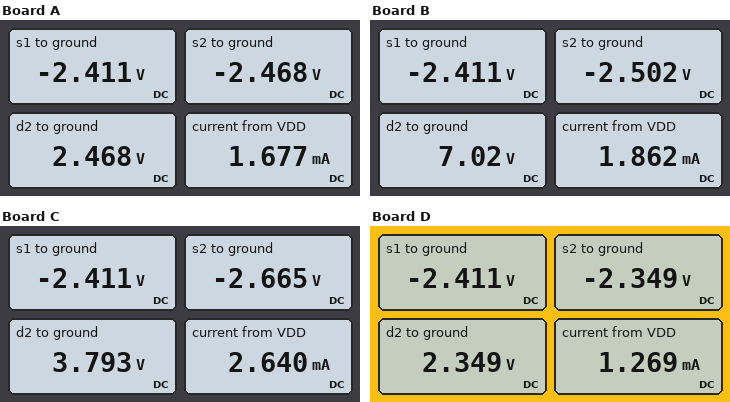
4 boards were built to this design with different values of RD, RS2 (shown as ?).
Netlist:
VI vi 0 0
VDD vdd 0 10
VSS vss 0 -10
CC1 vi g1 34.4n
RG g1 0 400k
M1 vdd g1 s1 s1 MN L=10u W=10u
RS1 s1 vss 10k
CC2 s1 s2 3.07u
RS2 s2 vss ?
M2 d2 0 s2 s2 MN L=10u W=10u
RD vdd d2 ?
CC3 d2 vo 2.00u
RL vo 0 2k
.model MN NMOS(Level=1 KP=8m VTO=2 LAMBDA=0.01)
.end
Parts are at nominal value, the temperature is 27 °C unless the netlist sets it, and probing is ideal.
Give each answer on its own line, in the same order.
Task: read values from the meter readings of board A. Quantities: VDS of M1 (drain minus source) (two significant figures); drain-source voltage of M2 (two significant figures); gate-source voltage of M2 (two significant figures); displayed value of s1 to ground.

12 V
4.9 V
2.5 V
-2.411 V
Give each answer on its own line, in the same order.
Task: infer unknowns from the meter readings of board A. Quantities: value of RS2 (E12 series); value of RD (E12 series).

8.2 kΩ
8.2 kΩ
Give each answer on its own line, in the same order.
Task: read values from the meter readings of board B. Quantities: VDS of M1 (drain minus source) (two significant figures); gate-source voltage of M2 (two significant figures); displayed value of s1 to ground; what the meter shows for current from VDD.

12 V
2.5 V
-2.411 V
1.862 mA
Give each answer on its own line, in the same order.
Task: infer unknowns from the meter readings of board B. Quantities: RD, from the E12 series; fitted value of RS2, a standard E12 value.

2.7 kΩ
6.8 kΩ
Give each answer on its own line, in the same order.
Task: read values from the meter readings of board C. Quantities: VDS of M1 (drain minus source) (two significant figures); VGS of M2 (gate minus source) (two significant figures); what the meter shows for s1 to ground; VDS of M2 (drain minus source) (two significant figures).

12 V
2.7 V
-2.411 V
6.5 V
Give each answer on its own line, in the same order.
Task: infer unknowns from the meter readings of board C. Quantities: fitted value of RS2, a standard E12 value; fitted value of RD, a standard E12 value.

3.9 kΩ
3.3 kΩ
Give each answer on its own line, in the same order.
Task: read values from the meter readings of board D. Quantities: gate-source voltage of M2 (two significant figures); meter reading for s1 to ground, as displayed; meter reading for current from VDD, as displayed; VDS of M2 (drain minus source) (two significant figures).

2.3 V
-2.411 V
1.269 mA
4.7 V
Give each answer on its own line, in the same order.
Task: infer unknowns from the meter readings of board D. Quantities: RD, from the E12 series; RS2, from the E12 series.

15 kΩ
15 kΩ
